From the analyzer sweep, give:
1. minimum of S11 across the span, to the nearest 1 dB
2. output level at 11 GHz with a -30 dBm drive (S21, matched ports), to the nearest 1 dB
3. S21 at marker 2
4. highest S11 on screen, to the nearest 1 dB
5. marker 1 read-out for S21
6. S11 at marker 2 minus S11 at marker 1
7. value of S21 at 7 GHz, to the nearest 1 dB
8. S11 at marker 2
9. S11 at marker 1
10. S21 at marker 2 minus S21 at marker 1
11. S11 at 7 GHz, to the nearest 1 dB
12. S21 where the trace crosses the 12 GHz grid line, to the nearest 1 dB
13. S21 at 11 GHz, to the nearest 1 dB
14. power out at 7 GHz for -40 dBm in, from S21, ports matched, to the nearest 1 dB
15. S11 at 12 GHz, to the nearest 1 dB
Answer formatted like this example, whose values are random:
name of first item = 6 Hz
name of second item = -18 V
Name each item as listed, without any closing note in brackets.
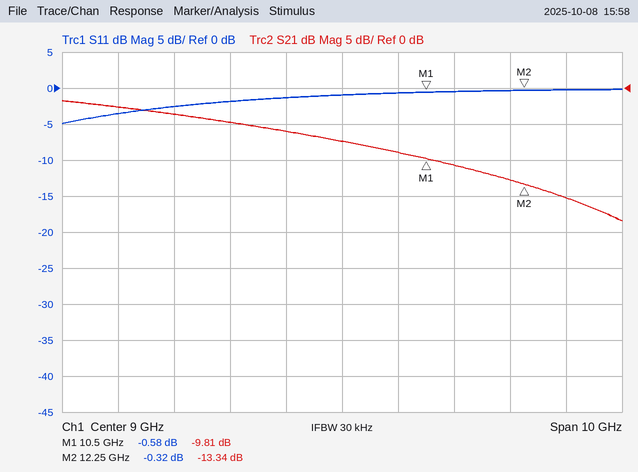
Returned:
minimum of S11 across the span, to the nearest 1 dB = -5 dB
output level at 11 GHz with a -30 dBm drive (S21, matched ports), to the nearest 1 dB = -41 dBm
S21 at marker 2 = -13.34 dB
highest S11 on screen, to the nearest 1 dB = 0 dB
marker 1 read-out for S21 = -9.81 dB
S11 at marker 2 minus S11 at marker 1 = 0.26 dB
value of S21 at 7 GHz, to the nearest 1 dB = -5 dB
S11 at marker 2 = -0.32 dB
S11 at marker 1 = -0.58 dB
S21 at marker 2 minus S21 at marker 1 = -3.53 dB
S11 at 7 GHz, to the nearest 1 dB = -2 dB
S21 where the trace crosses the 12 GHz grid line, to the nearest 1 dB = -13 dB
S21 at 11 GHz, to the nearest 1 dB = -11 dB
power out at 7 GHz for -40 dBm in, from S21, ports matched, to the nearest 1 dB = -45 dBm
S11 at 12 GHz, to the nearest 1 dB = 0 dB
